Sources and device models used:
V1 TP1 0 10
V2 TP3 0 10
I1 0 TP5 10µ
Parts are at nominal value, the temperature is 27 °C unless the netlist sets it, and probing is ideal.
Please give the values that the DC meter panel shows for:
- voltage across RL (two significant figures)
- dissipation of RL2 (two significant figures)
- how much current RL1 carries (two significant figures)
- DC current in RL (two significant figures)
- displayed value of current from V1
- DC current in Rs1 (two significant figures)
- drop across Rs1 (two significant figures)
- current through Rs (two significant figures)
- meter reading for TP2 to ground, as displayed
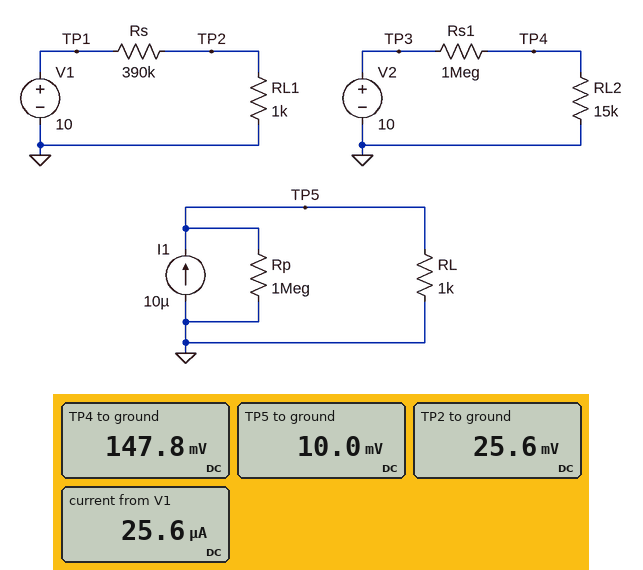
10 mV
1.5 µW
26 µA
10 µA
25.6 µA
9.9 µA
9.9 V
26 µA
25.6 mV
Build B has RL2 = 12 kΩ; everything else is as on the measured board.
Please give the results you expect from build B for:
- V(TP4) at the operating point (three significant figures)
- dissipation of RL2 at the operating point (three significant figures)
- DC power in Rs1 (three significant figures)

119 mV
1.17 µW
97.6 µW
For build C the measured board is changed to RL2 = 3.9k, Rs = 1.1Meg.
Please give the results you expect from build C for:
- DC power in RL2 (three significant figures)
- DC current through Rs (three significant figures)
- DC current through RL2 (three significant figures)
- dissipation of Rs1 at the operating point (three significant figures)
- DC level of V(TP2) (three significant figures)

387 nW
9.08 µA
9.96 µA
99.2 µW
9.08 mV
